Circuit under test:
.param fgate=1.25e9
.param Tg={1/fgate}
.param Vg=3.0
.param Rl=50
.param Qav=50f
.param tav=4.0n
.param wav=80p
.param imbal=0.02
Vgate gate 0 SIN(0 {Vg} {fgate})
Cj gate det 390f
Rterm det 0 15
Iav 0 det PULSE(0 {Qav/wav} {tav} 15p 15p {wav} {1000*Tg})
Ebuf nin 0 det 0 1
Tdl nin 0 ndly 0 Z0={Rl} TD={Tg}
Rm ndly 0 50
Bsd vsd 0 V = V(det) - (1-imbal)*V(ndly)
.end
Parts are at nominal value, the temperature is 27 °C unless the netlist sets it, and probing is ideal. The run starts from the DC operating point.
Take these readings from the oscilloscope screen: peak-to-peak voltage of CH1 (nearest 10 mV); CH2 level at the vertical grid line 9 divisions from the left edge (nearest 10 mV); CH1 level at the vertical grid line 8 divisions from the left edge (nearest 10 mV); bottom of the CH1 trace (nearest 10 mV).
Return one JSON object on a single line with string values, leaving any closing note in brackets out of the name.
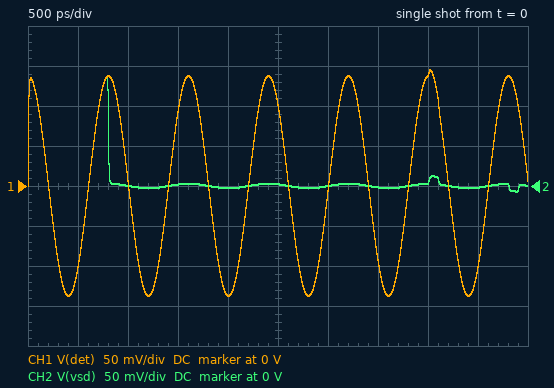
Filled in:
{"peak-to-peak voltage of CH1": "280 mV", "CH2 level at the vertical grid line 9 divisions from the left edge": "0 V", "CH1 level at the vertical grid line 8 divisions from the left edge": "140 mV", "bottom of the CH1 trace": "-140 mV"}
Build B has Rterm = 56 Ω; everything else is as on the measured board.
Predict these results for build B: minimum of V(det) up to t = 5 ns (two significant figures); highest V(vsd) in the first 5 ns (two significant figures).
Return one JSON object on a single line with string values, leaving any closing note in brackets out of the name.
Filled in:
{"minimum of V(det) up to t = 5 ns": "-510 mV", "highest V(vsd) in the first 5 ns": "500 mV"}
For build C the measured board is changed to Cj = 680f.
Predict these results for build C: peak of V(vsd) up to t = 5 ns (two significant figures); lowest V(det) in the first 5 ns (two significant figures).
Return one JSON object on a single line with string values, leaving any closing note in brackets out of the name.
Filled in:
{"peak of V(vsd) up to t = 5 ns": "240 mV", "lowest V(det) in the first 5 ns": "-240 mV"}
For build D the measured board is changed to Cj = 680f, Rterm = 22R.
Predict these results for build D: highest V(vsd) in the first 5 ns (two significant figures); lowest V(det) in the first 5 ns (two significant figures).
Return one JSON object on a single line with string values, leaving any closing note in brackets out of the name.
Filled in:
{"highest V(vsd) in the first 5 ns": "350 mV", "lowest V(det) in the first 5 ns": "-350 mV"}
